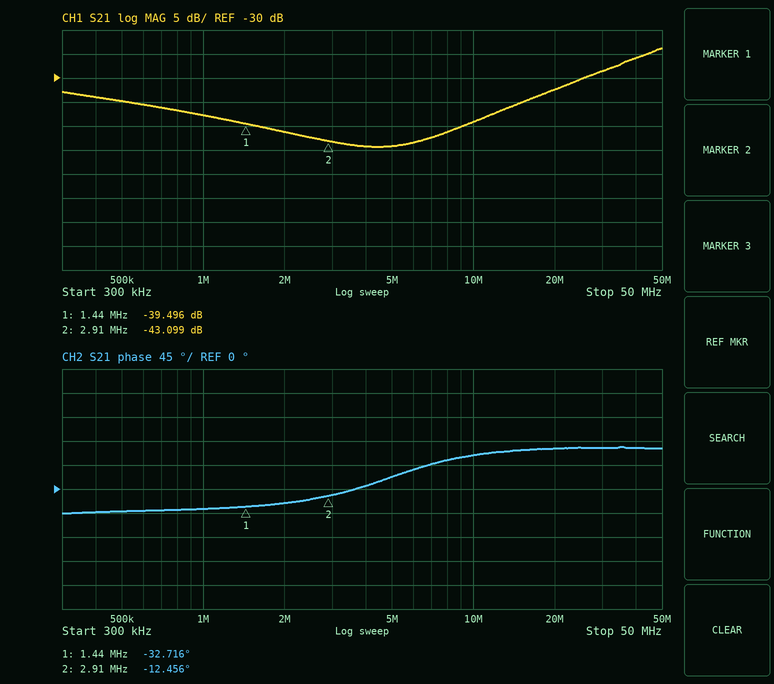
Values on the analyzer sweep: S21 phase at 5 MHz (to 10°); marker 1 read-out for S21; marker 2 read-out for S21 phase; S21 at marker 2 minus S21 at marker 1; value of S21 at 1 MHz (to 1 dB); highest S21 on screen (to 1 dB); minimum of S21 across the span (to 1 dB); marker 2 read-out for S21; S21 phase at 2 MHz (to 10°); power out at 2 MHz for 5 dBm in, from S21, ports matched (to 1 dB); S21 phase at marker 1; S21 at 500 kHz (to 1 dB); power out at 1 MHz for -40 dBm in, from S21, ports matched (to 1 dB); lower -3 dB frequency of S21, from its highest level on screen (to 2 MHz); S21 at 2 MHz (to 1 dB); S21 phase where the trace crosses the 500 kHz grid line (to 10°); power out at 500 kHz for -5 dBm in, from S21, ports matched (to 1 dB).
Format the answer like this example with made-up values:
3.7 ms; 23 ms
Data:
20°; -39.496 dB; -12.456°; -3.603 dB; -38 dB; -24 dB; -44 dB; -43.099 dB; -30°; -36 dBm; -32.716°; -35 dB; -78 dBm; 36 MHz; -41 dB; -40°; -40 dBm
